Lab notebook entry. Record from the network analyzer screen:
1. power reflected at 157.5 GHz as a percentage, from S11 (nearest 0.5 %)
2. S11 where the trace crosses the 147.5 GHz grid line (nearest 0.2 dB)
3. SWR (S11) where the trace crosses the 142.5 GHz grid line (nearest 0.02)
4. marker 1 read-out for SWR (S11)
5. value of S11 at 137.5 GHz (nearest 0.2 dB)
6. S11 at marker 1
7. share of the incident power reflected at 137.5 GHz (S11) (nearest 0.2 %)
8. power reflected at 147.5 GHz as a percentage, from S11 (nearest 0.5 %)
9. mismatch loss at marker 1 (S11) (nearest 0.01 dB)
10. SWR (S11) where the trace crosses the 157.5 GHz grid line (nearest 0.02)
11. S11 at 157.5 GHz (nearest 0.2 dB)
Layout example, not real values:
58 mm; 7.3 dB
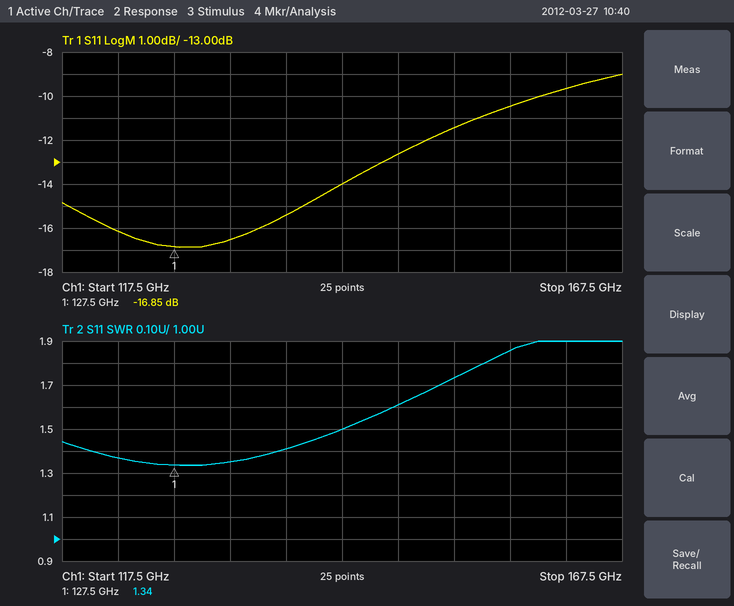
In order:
9.0 %; -12.6 dB; 1.50; 1.34; -15.4 dB; -16.85 dB; 2.8 %; 5.5 %; 0.09 dB; 1.86; -10.4 dB
